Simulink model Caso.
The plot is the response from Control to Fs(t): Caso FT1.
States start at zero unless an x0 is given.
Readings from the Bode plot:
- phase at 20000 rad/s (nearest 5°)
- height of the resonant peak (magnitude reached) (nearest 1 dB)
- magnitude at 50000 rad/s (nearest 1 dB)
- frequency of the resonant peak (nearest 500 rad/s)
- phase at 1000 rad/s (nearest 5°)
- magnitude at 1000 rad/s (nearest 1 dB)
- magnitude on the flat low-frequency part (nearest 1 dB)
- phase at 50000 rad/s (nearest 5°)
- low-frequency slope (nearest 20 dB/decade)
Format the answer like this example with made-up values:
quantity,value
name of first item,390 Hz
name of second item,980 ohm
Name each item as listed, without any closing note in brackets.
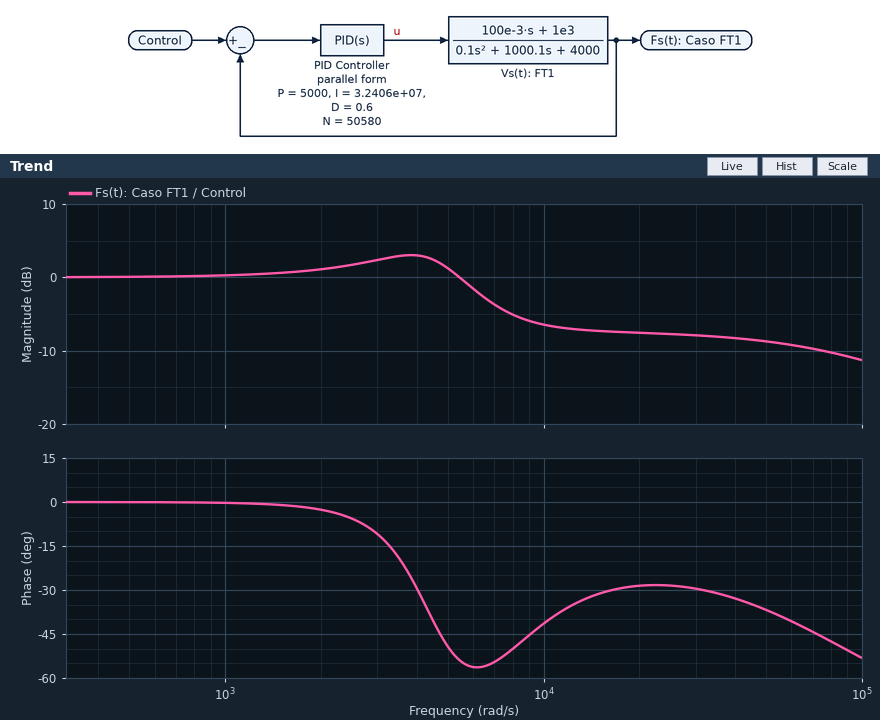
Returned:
quantity,value
phase at 20000 rad/s,-30°
height of the resonant peak (magnitude reached),3 dB
magnitude at 50000 rad/s,-9 dB
frequency of the resonant peak,4000 rad/s
phase at 1000 rad/s,0°
magnitude at 1000 rad/s,0 dB
magnitude on the flat low-frequency part,0 dB
phase at 50000 rad/s,-35°
low-frequency slope,0 dB/decade
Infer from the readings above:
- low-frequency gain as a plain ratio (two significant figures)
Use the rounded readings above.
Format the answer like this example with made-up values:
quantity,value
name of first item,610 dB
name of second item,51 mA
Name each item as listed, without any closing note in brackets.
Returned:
quantity,value
low-frequency gain as a plain ratio,1.0
